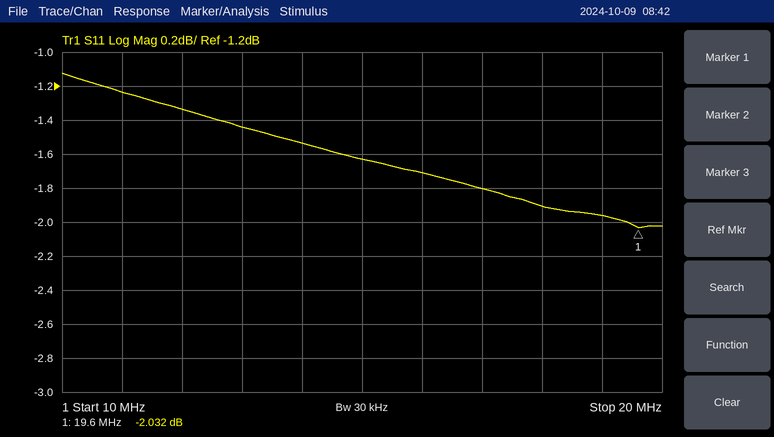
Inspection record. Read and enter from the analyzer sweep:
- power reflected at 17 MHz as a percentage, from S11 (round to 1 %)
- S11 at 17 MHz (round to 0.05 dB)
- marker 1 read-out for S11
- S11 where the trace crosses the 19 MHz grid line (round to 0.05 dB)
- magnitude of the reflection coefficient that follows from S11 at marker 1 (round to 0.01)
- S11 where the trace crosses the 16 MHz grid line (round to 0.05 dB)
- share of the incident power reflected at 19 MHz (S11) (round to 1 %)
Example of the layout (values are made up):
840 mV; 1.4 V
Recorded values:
66 %; -1.80 dB; -2.032 dB; -1.95 dB; 0.79; -1.70 dB; 64 %
